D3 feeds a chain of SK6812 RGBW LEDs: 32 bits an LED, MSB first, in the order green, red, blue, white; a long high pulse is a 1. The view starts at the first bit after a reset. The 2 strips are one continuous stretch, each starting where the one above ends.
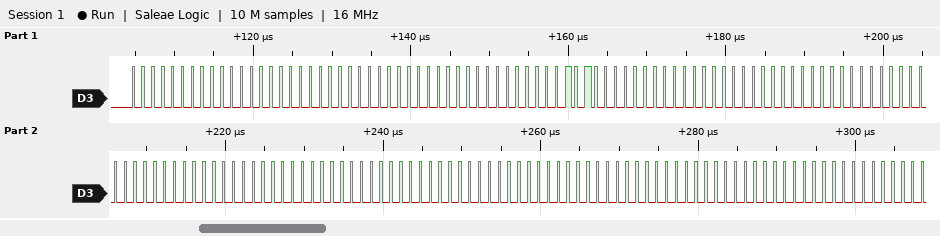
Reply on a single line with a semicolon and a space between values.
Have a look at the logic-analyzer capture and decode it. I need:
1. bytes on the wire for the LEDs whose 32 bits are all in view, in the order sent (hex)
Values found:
00 00 00 00 00 0A 00 00 00 00 00 00 00 00 00 00 00 00 00 00
